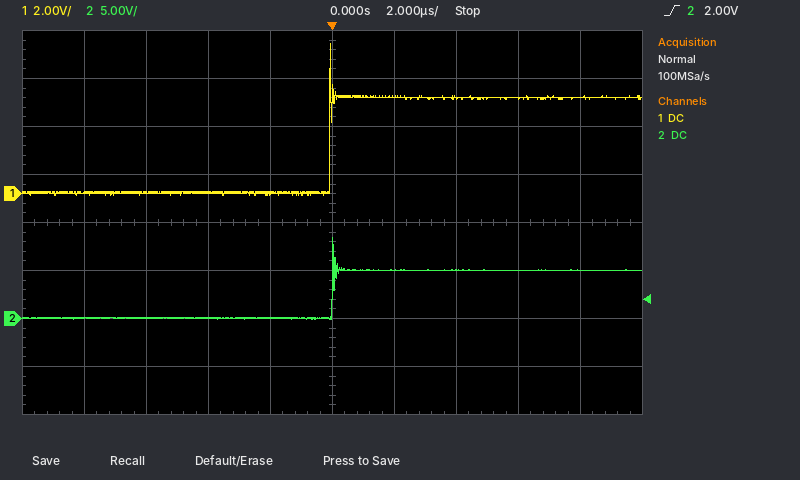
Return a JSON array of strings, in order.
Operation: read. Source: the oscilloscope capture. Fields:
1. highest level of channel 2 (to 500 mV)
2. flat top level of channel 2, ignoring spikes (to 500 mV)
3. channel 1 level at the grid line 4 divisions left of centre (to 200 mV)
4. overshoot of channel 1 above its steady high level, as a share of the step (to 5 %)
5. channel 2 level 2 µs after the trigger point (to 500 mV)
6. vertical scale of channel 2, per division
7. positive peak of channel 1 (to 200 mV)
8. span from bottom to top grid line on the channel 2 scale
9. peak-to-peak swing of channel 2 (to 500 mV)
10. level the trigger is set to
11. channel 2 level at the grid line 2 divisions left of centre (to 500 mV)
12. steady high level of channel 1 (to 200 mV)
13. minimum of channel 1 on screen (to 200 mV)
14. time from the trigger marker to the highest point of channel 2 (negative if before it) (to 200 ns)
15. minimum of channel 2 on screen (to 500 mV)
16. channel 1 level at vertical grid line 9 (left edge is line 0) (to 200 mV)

["8.5 V", "5.0 V", "0.0 V", "55 %", "5.0 V", "5 V", "6.2 V", "40 V", "8.5 V", "2.00 V", "0.0 V", "4.0 V", "0.0 V", "0.0 µs", "0.0 V", "4.0 V"]
